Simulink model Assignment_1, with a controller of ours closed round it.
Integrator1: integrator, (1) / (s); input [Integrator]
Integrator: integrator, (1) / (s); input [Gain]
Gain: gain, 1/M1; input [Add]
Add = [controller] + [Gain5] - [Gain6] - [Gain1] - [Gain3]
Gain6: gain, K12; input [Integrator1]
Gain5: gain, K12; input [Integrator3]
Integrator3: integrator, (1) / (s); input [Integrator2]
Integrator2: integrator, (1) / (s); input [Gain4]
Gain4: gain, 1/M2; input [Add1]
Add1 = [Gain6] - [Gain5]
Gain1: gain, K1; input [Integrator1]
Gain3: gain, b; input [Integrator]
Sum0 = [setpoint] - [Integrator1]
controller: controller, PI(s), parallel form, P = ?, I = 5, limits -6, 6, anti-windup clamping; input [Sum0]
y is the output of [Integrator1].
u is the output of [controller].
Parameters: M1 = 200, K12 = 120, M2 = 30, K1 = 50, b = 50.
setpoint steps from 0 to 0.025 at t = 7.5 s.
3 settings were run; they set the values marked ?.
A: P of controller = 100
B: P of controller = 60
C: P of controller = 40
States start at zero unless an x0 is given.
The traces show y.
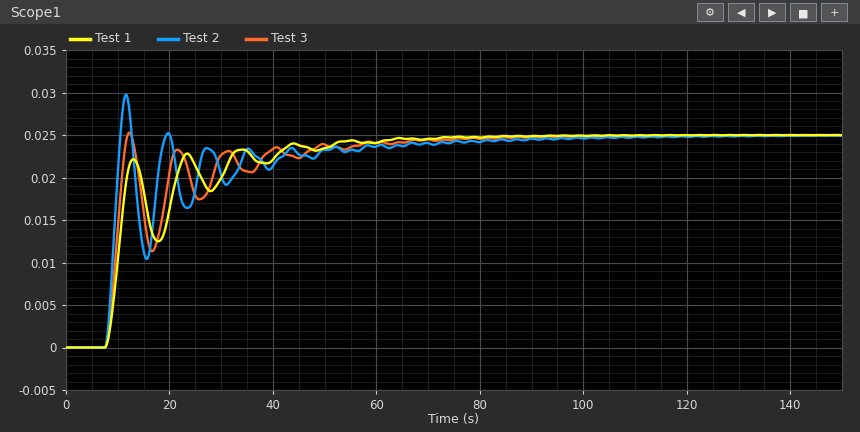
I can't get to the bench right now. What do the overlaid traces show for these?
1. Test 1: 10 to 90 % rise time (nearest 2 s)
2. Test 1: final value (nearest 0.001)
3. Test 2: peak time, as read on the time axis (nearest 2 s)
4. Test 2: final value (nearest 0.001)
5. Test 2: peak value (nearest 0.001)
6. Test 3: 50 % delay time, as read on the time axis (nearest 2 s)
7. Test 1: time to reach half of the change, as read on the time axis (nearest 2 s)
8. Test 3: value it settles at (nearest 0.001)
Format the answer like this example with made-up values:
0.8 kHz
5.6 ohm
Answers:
14 s
0.025
12 s
0.025
0.030
10 s
10 s
0.025
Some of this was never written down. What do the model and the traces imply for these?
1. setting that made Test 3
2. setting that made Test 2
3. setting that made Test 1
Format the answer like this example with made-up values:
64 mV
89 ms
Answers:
B
A
C
